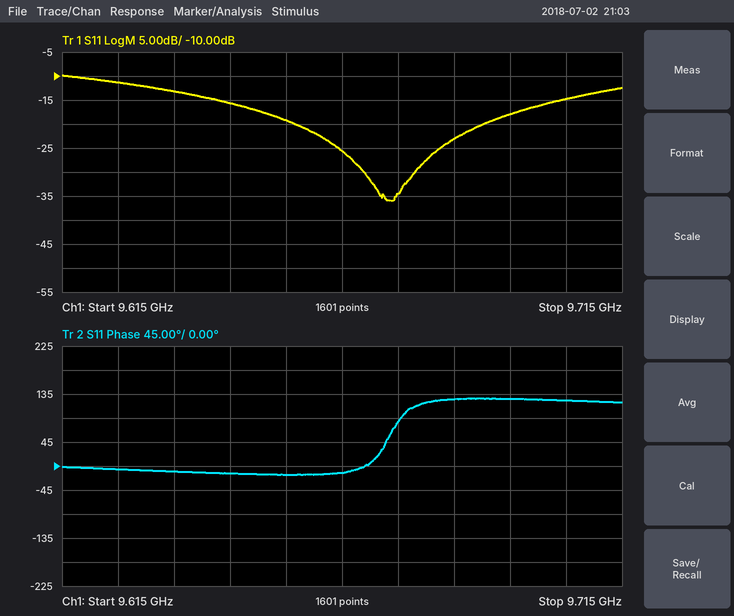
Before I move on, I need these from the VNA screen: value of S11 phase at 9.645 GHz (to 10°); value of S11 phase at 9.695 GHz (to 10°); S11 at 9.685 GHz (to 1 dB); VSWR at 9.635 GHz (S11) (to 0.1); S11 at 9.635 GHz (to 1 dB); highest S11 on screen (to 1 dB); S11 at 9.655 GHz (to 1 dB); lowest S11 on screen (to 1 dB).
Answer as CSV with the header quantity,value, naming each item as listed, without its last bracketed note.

quantity,value
value of S11 phase at 9.645 GHz,-10°
value of S11 phase at 9.695 GHz,130°
S11 at 9.685 GHz,-23 dB
VSWR at 9.635 GHz (S11),1.6
S11 at 9.635 GHz,-13 dB
highest S11 on screen,-10 dB
S11 at 9.655 GHz,-19 dB
lowest S11 on screen,-36 dB
